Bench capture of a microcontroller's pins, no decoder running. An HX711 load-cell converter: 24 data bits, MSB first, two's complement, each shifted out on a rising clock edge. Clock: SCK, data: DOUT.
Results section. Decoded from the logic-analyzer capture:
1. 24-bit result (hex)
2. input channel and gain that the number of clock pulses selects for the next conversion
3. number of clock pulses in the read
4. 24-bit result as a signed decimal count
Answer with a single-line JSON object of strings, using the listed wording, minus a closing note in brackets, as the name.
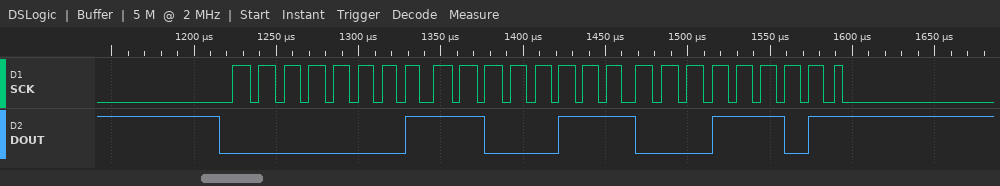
{"24-bit result": "0x01C71D", "input channel and gain that the number of clock pulses selects for the next conversion": "channel A, gain 128", "number of clock pulses in the read": "25", "24-bit result as a signed decimal count": "116509"}
